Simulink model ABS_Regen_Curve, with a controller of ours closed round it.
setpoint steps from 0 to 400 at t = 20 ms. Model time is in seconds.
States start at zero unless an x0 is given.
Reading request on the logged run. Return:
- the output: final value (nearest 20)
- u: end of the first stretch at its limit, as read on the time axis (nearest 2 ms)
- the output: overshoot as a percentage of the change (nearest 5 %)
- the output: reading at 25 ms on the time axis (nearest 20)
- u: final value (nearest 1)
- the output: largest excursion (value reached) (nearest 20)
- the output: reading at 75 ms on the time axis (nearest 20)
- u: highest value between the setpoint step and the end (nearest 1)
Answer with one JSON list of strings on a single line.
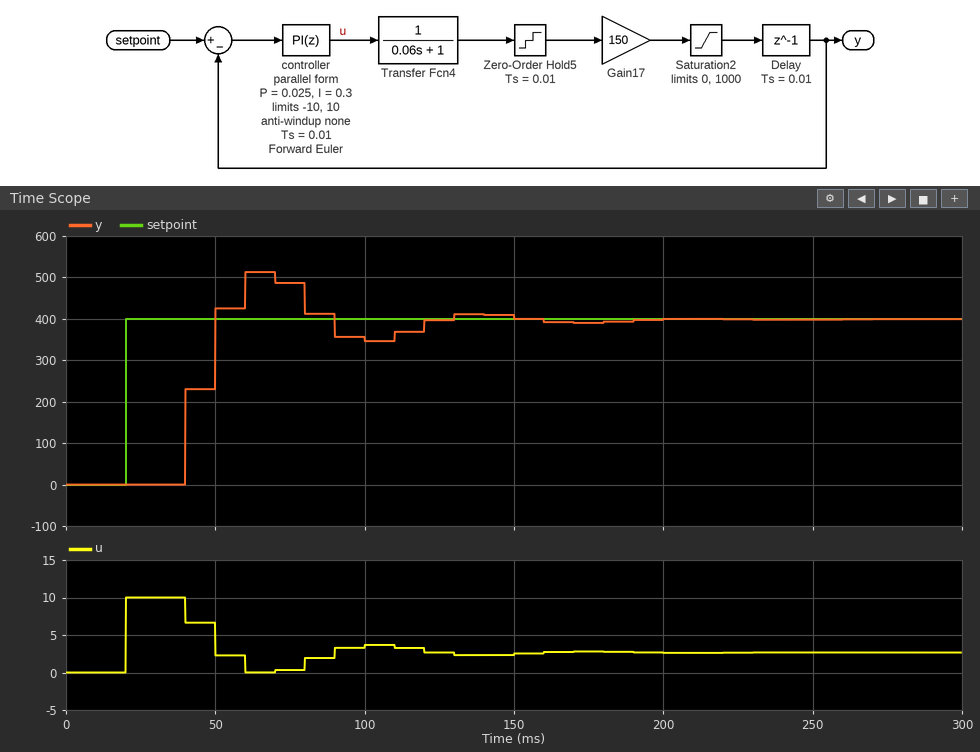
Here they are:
["400", "40 ms", "30 %", "0", "3", "520", "480", "10"]
